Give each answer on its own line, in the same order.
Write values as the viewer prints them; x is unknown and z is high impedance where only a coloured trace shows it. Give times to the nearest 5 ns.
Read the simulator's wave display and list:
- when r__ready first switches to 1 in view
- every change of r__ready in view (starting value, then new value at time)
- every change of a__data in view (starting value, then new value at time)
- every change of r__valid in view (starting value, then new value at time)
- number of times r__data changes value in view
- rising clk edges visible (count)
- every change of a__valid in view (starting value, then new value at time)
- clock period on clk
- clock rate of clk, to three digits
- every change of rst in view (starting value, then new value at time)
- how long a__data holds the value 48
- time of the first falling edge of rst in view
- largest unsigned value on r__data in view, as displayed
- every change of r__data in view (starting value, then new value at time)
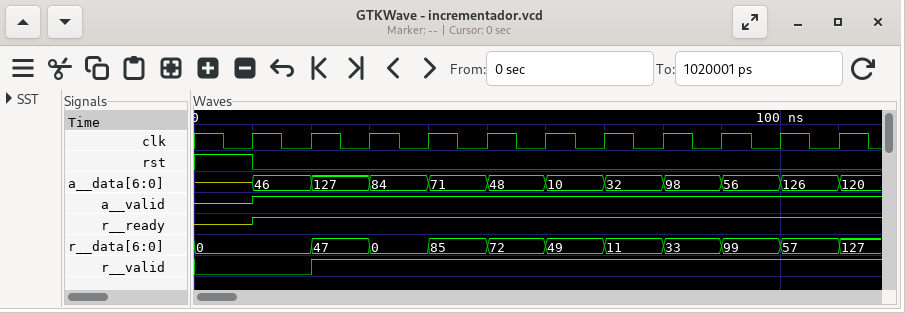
10 ns
z, 1 at 10 ns
z, 46 at 10 ns, 127 at 20 ns, 84 at 30 ns, 71 at 40 ns, 48 at 50 ns, 10 at 60 ns, 32 at 70 ns, 98 at 80 ns, 56 at 90 ns, 126 at 100 ns, 120 at 110 ns
0, 1 at 20 ns
10
11
z, 1 at 10 ns
10 ns
100 MHz
1, 0 at 10 ns
10 ns
10 ns
127
0, 47 at 20 ns, 0 at 30 ns, 85 at 40 ns, 72 at 50 ns, 49 at 60 ns, 11 at 70 ns, 33 at 80 ns, 99 at 90 ns, 57 at 100 ns, 127 at 110 ns
